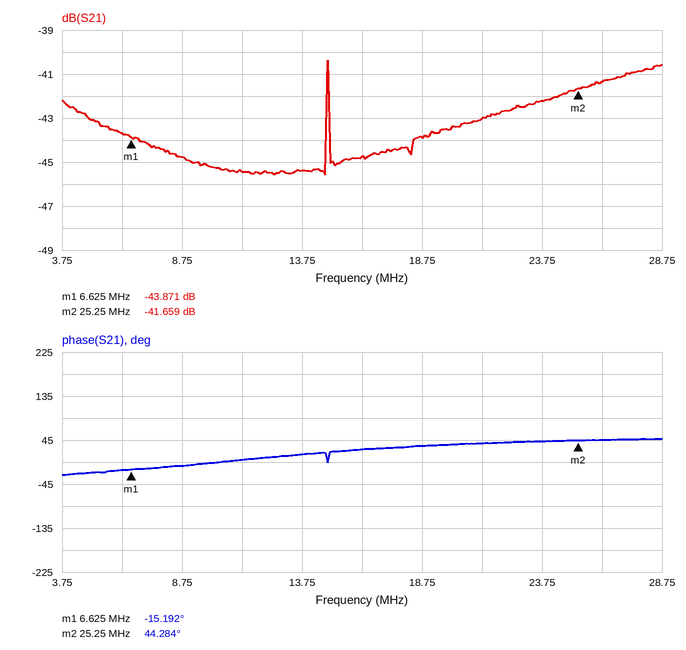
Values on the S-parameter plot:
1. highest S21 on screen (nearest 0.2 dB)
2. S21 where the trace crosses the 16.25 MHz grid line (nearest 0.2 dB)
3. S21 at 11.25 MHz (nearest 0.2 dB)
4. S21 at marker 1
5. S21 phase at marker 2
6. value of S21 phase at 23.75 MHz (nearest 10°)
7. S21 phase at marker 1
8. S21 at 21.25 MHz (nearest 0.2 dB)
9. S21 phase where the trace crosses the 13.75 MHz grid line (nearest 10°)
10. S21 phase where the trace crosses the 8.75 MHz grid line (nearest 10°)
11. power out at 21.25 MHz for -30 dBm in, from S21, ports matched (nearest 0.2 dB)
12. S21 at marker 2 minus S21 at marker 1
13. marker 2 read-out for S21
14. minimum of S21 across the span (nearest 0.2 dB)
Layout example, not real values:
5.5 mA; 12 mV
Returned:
-40.4 dB; -44.8 dB; -45.4 dB; -43.871 dB; 44.284°; 40°; -15.192°; -43.0 dB; 20°; -10°; -73.0 dBm; 2.212 dB; -41.659 dB; -45.6 dB
